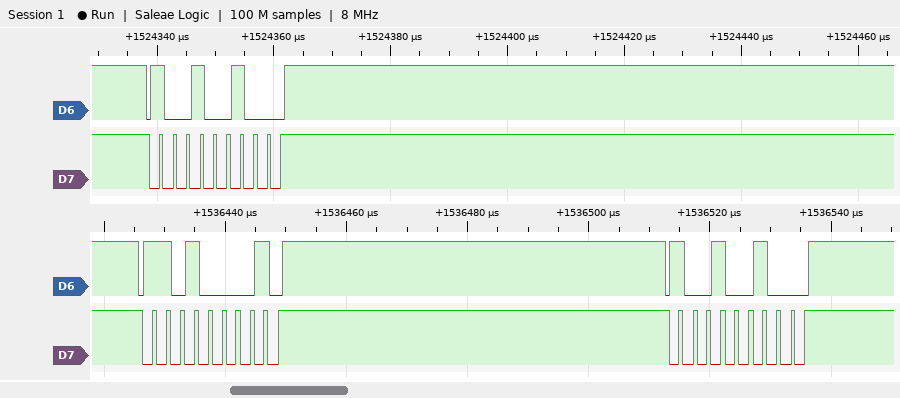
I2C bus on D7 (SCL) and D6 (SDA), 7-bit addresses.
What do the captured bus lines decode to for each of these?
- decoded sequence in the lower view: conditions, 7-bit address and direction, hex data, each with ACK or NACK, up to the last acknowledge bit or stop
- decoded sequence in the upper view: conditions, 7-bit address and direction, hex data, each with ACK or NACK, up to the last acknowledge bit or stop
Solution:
start, address 68 write NACK, stop, start, address 49 write ACK, stop
start, address 49 write ACK, stop
